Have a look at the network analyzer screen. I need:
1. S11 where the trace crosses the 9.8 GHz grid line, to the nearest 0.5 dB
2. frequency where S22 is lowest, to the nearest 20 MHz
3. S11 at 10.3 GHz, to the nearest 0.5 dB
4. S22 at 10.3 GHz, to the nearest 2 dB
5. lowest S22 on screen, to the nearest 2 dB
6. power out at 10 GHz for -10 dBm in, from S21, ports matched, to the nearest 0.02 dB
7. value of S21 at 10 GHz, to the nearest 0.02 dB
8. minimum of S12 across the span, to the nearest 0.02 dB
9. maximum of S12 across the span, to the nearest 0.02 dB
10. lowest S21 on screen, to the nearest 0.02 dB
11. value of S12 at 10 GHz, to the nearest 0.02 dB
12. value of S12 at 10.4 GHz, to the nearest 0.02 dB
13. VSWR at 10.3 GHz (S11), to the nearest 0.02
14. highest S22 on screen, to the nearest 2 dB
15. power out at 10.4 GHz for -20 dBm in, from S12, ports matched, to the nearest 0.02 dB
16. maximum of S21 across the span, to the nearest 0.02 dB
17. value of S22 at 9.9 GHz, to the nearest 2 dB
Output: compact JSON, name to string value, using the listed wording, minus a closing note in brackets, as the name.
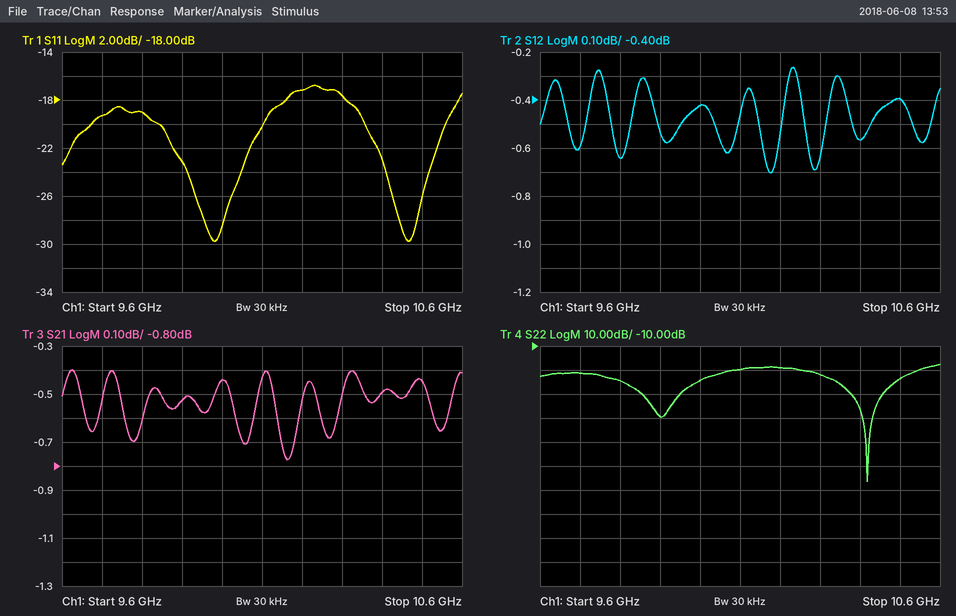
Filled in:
{"S11 where the trace crosses the 9.8 GHz grid line, to the nearest 0.5 dB": "-19.0 dB", "frequency where S22 is lowest, to the nearest 20 MHz": "10.42 GHz", "S11 at 10.3 GHz, to the nearest 0.5 dB": "-17.5 dB", "S22 at 10.3 GHz, to the nearest 2 dB": "-22 dB", "lowest S22 on screen, to the nearest 2 dB": "-66 dB", "power out at 10 GHz for -10 dBm in, from S21, ports matched, to the nearest 0.02 dB": "-10.44 dBm", "value of S21 at 10 GHz, to the nearest 0.02 dB": "-0.44 dB", "minimum of S12 across the span, to the nearest 0.02 dB": "-0.70 dB", "maximum of S12 across the span, to the nearest 0.02 dB": "-0.26 dB", "lowest S21 on screen, to the nearest 0.02 dB": "-0.78 dB", "value of S12 at 10 GHz, to the nearest 0.02 dB": "-0.42 dB", "value of S12 at 10.4 GHz, to the nearest 0.02 dB": "-0.56 dB", "VSWR at 10.3 GHz (S11), to the nearest 0.02": "1.30", "highest S22 on screen, to the nearest 2 dB": "-18 dB", "power out at 10.4 GHz for -20 dBm in, from S12, ports matched, to the nearest 0.02 dB": "-20.56 dBm", "maximum of S21 across the span, to the nearest 0.02 dB": "-0.40 dB", "value of S22 at 9.9 GHz, to the nearest 2 dB": "-40 dB"}
